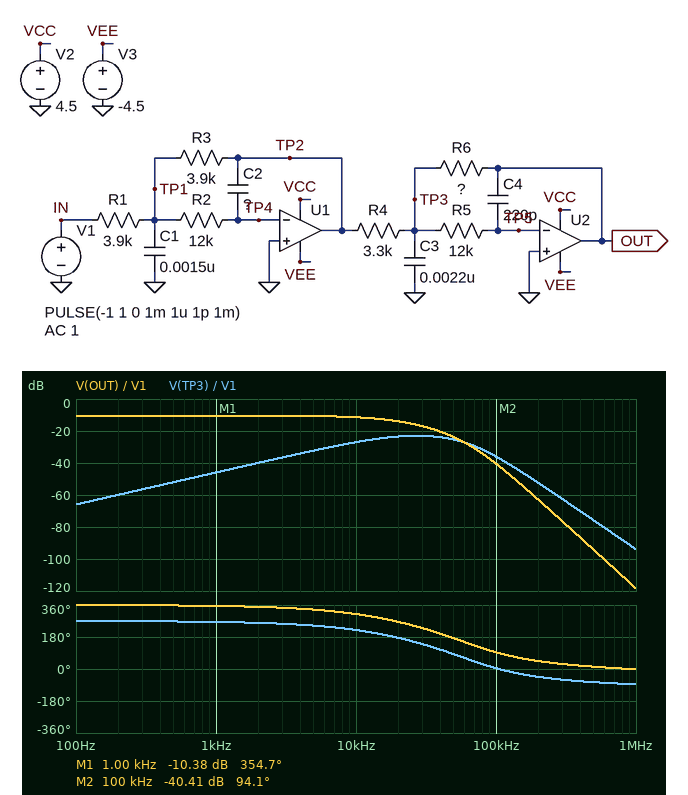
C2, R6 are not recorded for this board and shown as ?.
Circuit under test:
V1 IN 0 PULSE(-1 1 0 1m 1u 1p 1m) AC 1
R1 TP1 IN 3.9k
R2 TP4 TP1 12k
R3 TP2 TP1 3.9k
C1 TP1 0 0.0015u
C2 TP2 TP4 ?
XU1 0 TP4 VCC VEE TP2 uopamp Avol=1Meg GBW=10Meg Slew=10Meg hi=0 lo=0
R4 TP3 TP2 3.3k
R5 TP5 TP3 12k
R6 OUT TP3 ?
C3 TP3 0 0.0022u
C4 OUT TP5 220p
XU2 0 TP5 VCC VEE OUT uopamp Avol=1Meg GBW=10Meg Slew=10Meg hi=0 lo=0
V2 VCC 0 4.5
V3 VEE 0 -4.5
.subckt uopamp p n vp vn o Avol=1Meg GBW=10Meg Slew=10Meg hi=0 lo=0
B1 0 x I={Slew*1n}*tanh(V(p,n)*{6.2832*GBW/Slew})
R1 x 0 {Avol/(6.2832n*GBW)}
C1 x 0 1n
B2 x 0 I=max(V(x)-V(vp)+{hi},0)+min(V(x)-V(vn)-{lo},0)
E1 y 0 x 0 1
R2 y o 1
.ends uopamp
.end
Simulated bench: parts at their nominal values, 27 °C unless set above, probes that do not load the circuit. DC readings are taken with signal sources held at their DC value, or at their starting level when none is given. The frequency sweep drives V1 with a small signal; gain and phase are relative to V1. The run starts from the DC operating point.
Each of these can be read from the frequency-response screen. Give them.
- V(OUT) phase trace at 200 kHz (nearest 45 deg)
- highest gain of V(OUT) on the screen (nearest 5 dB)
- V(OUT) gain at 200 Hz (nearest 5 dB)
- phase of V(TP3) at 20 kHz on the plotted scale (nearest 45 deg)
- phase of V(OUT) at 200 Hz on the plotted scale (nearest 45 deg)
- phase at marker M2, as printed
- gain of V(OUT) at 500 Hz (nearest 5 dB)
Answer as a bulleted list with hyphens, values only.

- 45 deg
- -10 dB
- -10 dB
- 180 deg
- 360 deg
- 94.1 deg
- -10 dB
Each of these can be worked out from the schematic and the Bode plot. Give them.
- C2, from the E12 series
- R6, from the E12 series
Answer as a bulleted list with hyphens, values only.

- 390 pF
- 1 kΩ
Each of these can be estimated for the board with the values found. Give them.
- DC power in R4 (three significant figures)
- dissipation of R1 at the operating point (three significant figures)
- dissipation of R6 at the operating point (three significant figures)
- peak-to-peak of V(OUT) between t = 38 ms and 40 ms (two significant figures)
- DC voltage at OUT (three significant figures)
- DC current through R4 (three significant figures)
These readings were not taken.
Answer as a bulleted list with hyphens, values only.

- 303 µW
- 256 µW
- 91.8 µW
- 580 mV
- -303 mV
- 303 µA
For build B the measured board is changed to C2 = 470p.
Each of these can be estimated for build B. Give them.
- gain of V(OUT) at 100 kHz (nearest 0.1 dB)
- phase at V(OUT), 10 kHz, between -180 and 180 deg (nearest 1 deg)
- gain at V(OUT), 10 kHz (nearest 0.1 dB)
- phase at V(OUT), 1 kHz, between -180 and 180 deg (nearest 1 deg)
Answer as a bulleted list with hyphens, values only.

- -42.1 dB
- -57 deg
- -12.0 dB
- -6 deg
